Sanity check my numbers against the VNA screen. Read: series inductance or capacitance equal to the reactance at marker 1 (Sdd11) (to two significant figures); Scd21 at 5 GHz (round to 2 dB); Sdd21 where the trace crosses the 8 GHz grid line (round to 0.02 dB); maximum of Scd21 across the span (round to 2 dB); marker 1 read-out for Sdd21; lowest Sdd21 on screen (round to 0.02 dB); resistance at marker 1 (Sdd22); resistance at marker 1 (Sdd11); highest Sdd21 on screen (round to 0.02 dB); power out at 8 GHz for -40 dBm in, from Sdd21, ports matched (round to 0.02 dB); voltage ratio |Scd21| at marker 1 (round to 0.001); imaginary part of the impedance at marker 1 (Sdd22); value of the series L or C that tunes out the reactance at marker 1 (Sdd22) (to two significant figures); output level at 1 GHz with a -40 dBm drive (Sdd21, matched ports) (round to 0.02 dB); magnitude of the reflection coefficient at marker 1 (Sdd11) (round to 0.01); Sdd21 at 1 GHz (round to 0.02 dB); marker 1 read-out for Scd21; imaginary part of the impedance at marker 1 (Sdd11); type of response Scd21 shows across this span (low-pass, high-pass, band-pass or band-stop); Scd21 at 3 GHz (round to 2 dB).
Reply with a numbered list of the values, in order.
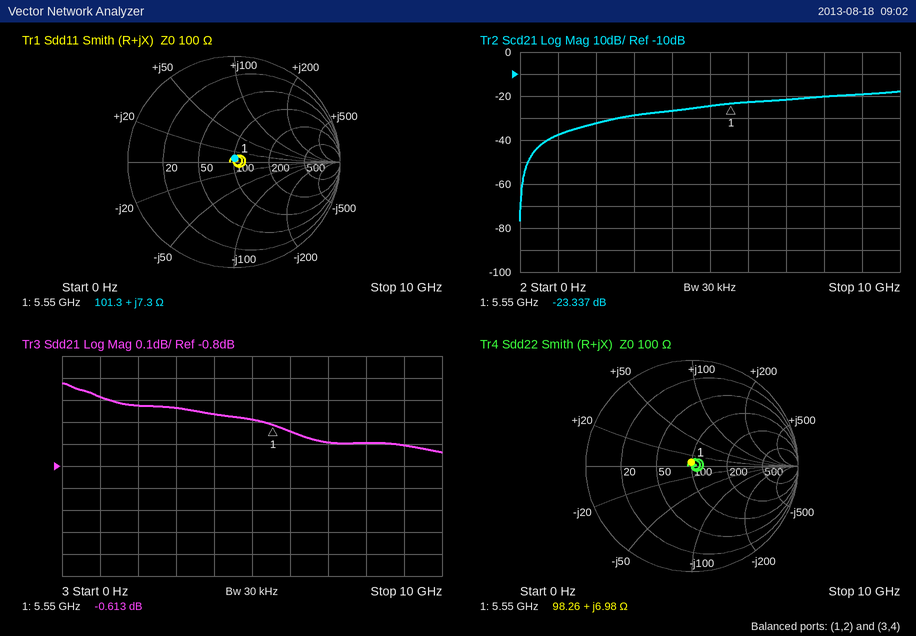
1. 210 pH
2. -24 dB
3. -0.70 dB
4. -18 dB
5. -0.613 dB
6. -0.74 dB
7. 98.26 Ω
8. 101.3 Ω
9. -0.42 dB
10. -40.70 dBm
11. 0.068
12. +6.98 Ω
13. 4.1 pF
14. -40.48 dBm
15. 0.04
16. -0.48 dB
17. -23.337 dB
18. +7.3 Ω
19. high-pass
20. -28 dB
